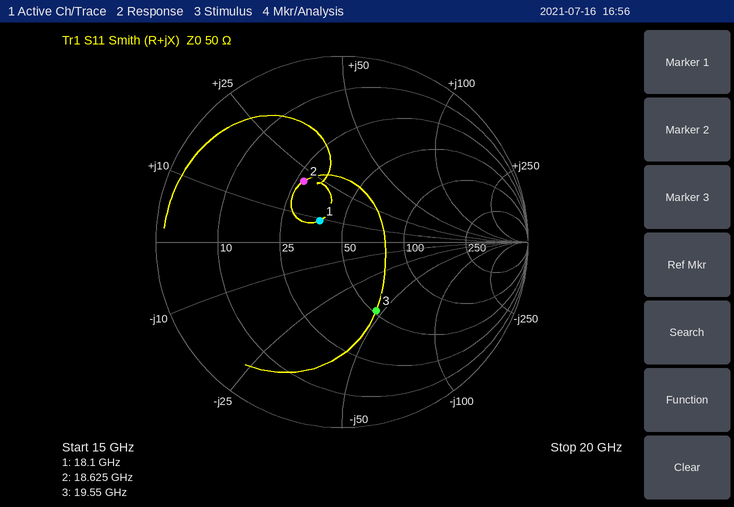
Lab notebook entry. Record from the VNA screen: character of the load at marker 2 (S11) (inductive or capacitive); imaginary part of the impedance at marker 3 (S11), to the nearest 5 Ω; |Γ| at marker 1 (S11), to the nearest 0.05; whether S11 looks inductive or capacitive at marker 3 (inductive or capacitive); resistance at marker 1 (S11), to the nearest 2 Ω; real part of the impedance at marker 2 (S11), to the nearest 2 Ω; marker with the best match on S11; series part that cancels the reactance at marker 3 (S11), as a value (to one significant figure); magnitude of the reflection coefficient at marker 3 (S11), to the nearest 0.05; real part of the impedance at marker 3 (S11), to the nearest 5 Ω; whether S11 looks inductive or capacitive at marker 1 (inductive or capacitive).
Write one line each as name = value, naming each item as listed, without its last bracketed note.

character of the load at marker 2 (S11) = inductive
imaginary part of the impedance at marker 3 (S11), to the nearest 5 Ω = -45 Ω
|Γ| at marker 1 (S11), to the nearest 0.05 = 0.15
whether S11 looks inductive or capacitive at marker 3 = capacitive
resistance at marker 1 (S11), to the nearest 2 Ω = 38 Ω
real part of the impedance at marker 2 (S11), to the nearest 2 Ω = 28 Ω
marker with the best match on S11 = marker 1
series part that cancels the reactance at marker 3 (S11), as a value = 400 pH
magnitude of the reflection coefficient at marker 3 (S11), to the nearest 0.05 = 0.40
real part of the impedance at marker 3 (S11), to the nearest 5 Ω = 50 Ω
whether S11 looks inductive or capacitive at marker 1 = inductive
